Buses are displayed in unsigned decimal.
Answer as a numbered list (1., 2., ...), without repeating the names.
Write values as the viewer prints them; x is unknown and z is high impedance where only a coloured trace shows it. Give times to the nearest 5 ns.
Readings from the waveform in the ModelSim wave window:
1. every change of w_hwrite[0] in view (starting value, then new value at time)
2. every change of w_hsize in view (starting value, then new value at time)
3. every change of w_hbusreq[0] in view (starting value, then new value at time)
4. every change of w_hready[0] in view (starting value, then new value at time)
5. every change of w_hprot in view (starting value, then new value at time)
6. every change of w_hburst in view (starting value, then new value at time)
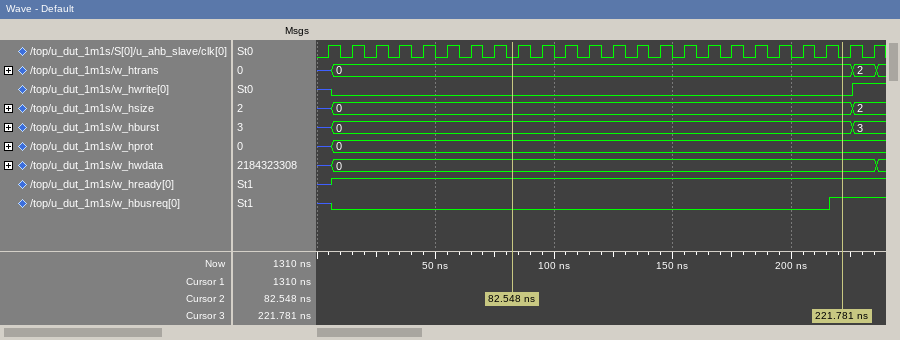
1. z, 0 at 5 ns, 1 at 225 ns
2. z, 0 at 5 ns, 2 at 225 ns
3. z, 0 at 5 ns, 1 at 215 ns
4. z, 1 at 5 ns
5. z, 0 at 5 ns
6. z, 0 at 5 ns, 3 at 225 ns
